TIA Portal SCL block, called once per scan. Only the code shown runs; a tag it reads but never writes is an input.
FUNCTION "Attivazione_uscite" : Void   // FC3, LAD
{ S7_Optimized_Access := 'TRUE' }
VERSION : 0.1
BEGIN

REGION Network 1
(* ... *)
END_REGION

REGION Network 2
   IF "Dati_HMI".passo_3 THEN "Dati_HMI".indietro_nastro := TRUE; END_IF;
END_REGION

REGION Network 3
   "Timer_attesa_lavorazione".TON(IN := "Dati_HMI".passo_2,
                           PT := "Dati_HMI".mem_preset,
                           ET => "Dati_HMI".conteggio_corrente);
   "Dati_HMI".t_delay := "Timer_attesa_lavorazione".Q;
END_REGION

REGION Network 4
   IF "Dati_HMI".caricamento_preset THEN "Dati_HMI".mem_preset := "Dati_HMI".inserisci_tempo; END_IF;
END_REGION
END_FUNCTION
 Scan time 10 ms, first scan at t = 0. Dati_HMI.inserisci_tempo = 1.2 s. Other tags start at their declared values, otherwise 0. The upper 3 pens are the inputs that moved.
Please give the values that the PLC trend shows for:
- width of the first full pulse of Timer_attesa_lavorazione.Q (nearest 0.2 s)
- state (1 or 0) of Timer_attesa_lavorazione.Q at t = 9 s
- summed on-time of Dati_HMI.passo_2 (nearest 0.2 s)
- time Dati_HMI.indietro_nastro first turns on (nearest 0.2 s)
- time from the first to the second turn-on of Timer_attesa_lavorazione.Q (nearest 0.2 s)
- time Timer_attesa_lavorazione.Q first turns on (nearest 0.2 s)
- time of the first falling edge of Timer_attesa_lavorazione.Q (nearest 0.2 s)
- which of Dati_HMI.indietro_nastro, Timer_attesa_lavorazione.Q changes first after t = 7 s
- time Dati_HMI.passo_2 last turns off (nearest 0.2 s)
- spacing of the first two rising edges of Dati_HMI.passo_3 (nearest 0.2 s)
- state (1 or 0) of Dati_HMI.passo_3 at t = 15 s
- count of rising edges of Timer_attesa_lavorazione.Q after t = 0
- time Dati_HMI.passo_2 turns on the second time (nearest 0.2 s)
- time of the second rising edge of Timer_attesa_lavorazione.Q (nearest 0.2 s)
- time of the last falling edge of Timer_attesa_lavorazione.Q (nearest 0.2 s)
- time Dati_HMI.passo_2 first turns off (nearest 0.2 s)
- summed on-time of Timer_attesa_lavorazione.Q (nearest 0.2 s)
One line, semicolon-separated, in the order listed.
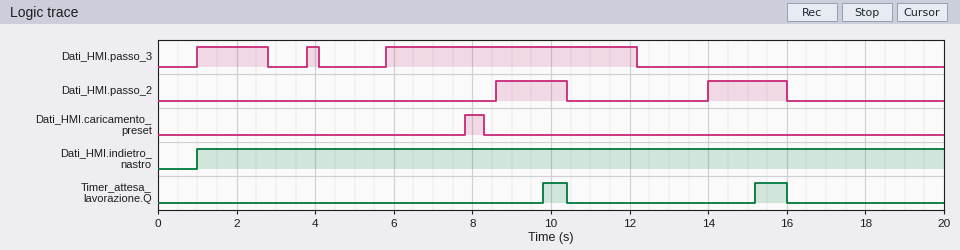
0.6 s; 0; 3.8 s; 1.0 s; 5.4 s; 9.8 s; 10.4 s; Timer_attesa_lavorazione.Q; 16.0 s; 2.8 s; 0; 2; 14.0 s; 15.2 s; 16.0 s; 10.4 s; 1.4 s
